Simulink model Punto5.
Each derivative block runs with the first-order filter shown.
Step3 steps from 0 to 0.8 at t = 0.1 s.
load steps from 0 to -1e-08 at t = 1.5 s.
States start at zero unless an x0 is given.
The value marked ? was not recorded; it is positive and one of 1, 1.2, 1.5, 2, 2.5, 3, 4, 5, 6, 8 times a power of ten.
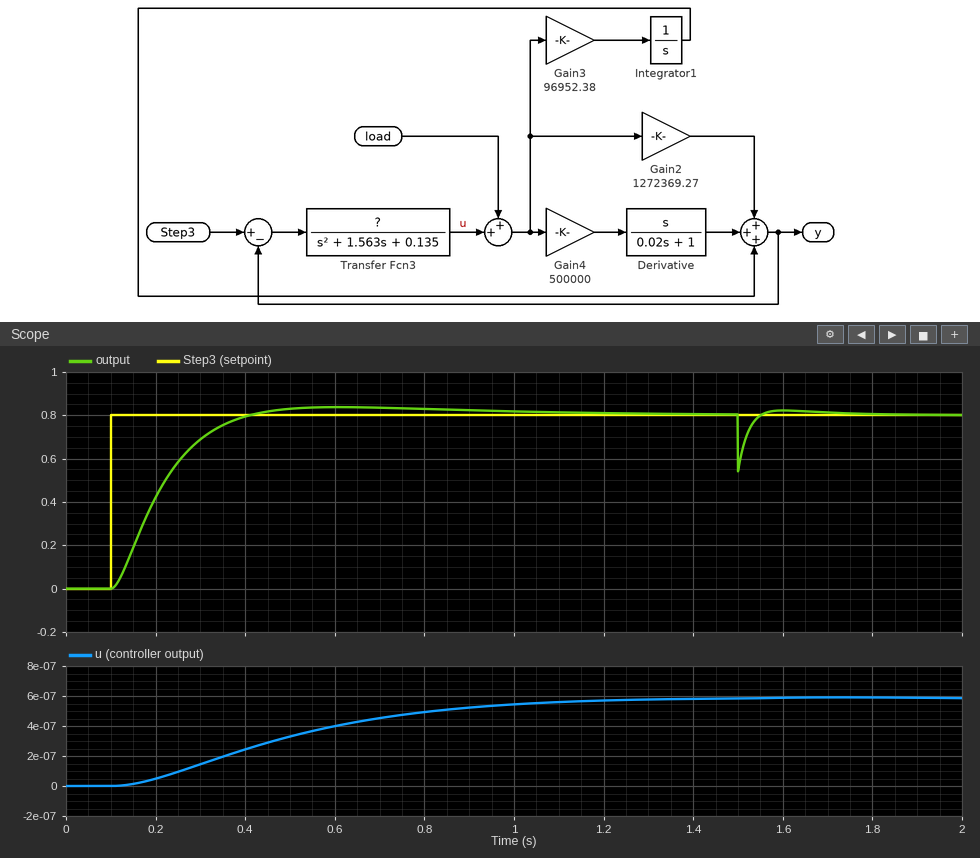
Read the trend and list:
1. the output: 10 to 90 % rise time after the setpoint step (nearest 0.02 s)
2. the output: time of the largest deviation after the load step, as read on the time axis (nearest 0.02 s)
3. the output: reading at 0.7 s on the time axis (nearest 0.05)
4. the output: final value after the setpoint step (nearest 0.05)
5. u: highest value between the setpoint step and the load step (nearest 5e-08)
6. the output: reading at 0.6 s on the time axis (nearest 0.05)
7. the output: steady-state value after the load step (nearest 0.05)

0.20 s
1.50 s
0.85
0.80
0.00000060
0.85
0.80
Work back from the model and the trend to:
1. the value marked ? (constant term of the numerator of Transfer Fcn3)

1.5e-05
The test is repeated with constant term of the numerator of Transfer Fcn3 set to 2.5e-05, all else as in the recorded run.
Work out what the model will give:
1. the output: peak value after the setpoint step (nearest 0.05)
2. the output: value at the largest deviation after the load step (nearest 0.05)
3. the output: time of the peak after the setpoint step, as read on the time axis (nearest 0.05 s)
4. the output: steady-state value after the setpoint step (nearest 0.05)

0.85
0.55
0.40 s
0.80
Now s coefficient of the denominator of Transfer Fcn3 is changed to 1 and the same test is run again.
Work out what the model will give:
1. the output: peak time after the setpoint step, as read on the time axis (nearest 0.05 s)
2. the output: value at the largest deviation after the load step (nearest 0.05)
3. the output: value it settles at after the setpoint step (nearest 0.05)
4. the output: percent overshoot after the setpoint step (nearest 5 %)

0.55 s
0.55
0.80
10 %
